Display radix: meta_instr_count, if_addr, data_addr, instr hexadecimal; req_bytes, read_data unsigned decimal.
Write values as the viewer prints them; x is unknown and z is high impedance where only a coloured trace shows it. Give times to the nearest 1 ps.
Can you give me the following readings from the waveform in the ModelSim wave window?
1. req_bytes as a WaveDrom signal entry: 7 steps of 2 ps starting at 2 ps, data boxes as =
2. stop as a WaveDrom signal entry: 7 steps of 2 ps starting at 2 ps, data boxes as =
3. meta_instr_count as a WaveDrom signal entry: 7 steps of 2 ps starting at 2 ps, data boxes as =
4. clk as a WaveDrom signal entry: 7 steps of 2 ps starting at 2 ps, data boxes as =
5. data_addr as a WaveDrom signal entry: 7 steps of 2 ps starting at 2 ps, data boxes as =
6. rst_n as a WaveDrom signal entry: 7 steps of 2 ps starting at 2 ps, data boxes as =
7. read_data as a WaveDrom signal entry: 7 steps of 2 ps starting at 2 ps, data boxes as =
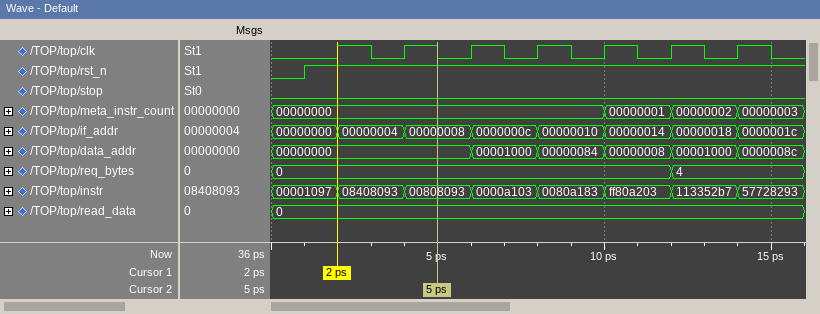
{name: 'req_bytes', wave: '=....=.', data: '0 4'}
{name: 'stop', wave: '0......'}
{name: 'meta_instr_count', wave: '=...===', data: '00000000 00000001 00000002 00000003'}
{name: 'clk', wave: 'p......'}
{name: 'data_addr', wave: '=.=====', data: '00000000 00001000 00000084 00000008 00001000 0000008c'}
{name: 'rst_n', wave: '1......'}
{name: 'read_data', wave: '=......', data: '0'}
